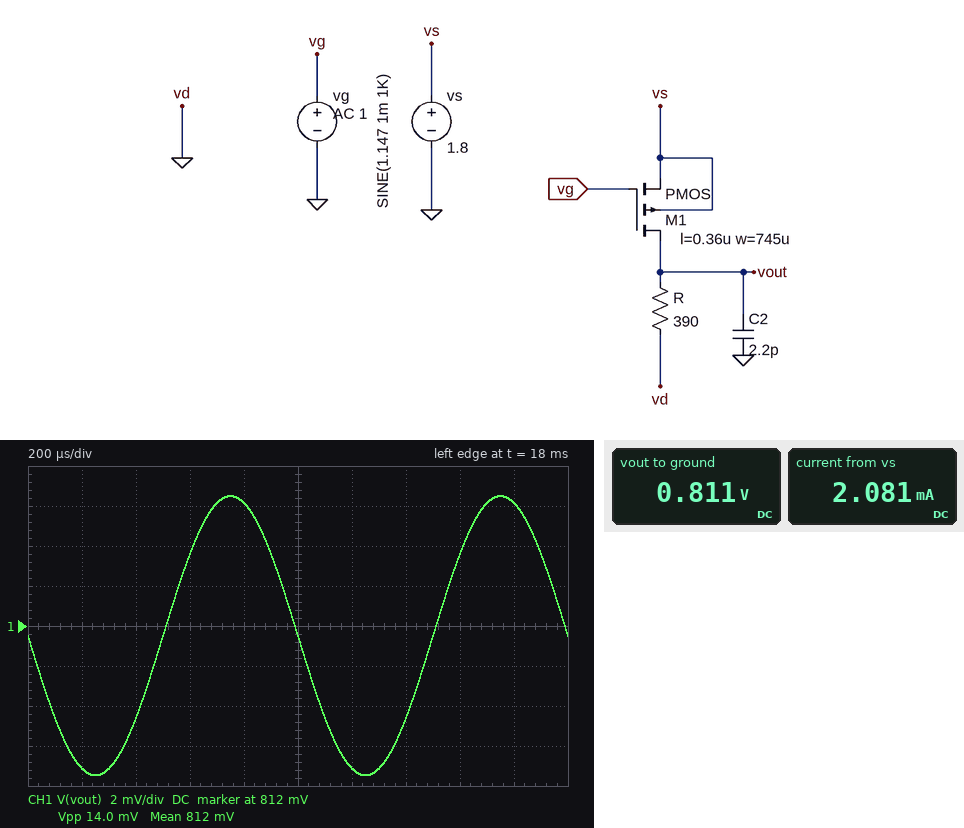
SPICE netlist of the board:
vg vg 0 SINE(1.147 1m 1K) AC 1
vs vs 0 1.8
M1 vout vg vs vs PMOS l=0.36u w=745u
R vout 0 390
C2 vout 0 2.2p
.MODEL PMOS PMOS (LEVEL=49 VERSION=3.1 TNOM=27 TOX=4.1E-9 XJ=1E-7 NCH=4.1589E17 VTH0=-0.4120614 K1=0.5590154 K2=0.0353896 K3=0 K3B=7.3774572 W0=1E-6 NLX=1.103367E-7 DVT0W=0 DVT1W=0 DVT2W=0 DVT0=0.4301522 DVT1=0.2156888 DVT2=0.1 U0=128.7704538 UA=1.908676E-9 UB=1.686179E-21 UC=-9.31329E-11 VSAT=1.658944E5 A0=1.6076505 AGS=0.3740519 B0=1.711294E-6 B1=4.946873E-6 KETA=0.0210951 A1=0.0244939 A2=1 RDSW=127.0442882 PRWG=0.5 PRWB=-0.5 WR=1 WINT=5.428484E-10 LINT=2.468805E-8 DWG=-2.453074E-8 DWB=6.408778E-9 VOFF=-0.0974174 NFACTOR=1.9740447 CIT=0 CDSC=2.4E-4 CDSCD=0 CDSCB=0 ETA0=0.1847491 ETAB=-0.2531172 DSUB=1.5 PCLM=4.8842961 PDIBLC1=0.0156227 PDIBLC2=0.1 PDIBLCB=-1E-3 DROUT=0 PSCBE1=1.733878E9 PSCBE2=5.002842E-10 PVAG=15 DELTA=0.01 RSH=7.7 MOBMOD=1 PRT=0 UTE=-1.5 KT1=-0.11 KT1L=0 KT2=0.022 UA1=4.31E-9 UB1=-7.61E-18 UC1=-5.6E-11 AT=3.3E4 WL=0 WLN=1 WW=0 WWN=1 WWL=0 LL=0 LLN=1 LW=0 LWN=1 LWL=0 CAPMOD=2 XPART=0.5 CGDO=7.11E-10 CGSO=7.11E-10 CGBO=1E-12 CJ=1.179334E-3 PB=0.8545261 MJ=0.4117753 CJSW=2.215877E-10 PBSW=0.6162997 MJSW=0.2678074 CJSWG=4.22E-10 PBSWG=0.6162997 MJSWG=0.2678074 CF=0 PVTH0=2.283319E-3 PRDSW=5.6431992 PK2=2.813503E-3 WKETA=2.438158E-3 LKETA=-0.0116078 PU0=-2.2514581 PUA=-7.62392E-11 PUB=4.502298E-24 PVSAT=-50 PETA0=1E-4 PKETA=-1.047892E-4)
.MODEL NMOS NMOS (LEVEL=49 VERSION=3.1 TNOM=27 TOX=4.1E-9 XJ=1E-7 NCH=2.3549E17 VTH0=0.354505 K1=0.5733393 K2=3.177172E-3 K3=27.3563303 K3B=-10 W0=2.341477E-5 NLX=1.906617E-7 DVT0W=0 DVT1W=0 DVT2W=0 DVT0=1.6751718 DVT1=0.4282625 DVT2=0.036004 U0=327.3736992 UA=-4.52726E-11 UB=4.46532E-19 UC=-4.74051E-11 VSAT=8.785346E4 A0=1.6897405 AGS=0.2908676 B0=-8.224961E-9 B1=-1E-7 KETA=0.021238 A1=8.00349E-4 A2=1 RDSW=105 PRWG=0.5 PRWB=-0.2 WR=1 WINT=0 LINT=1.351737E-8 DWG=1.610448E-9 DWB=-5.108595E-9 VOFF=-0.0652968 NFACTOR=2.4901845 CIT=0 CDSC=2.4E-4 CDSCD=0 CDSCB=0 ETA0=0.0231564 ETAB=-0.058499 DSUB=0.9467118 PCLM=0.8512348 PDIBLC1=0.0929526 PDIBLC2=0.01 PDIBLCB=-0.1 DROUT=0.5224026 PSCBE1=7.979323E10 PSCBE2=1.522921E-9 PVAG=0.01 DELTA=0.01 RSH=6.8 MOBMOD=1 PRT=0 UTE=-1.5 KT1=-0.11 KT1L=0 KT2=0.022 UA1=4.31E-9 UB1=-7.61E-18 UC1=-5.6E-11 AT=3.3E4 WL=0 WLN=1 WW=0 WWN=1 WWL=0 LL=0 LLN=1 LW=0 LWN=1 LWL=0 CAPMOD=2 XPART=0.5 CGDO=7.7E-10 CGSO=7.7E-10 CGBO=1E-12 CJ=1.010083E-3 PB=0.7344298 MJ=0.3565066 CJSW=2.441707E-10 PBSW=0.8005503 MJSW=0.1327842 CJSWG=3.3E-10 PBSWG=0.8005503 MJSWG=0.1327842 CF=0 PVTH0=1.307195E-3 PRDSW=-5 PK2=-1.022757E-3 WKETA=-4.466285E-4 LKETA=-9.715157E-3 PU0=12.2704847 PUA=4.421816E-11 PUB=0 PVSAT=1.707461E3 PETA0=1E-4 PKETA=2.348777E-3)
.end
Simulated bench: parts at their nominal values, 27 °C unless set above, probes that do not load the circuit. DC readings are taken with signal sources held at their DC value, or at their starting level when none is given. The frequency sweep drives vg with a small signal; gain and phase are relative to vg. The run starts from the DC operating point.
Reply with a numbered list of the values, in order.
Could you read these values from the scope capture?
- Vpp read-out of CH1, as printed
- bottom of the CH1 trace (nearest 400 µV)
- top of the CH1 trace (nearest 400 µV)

1. 14.0 mV
2. 804.4 mV
3. 818.4 mV
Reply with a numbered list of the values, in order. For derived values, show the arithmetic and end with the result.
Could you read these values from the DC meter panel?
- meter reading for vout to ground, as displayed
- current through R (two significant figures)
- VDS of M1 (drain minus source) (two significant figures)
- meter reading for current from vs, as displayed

1. 0.811 V
2. (811 mV) / 390 Ω = 2.1 mA
3. 811 mV - 1.8 V = -990 mV
4. 2.081 mA
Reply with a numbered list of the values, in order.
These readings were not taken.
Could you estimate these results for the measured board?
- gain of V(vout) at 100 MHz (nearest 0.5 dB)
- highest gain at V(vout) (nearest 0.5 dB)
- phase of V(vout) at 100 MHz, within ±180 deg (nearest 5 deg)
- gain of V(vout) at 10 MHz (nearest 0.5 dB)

1. 15.0 dB
2. 17.0 dB
3. 145 deg
4. 17.0 dB
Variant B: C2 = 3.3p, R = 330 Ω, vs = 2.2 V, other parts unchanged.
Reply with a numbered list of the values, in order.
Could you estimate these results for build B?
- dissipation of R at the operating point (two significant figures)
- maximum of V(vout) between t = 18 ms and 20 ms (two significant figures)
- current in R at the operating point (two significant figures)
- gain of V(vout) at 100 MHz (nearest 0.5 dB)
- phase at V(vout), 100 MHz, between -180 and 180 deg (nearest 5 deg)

1. 12 mW
2. 2.0 V
3. 6.1 mA
4. -15.0 dB
5. 165 deg
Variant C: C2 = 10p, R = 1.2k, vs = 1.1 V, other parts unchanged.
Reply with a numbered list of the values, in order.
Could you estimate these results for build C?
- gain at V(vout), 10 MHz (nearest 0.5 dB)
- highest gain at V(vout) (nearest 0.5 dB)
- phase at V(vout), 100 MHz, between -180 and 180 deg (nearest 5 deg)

1. -30.0 dB
2. -26.0 dB
3. 5 deg
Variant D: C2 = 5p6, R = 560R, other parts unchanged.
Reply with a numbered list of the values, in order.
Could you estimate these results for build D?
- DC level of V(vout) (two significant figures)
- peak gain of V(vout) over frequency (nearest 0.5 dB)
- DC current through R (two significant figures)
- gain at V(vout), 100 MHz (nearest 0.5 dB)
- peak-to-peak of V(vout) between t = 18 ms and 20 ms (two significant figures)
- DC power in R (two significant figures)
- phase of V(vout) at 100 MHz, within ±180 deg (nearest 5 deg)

1. 1.1 V
2. 19.5 dB
3. 2.0 mA
4. 12.5 dB
5. 19 mV
6. 2.3 mW
7. 115 deg
